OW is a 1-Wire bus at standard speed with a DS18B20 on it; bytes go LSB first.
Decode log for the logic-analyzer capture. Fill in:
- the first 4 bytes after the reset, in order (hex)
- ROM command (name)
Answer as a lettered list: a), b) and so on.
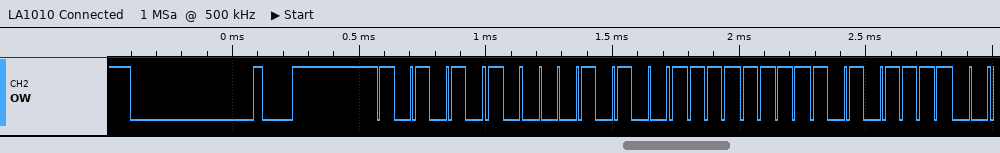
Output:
a) 55 28 FF F5
b) Match ROM
